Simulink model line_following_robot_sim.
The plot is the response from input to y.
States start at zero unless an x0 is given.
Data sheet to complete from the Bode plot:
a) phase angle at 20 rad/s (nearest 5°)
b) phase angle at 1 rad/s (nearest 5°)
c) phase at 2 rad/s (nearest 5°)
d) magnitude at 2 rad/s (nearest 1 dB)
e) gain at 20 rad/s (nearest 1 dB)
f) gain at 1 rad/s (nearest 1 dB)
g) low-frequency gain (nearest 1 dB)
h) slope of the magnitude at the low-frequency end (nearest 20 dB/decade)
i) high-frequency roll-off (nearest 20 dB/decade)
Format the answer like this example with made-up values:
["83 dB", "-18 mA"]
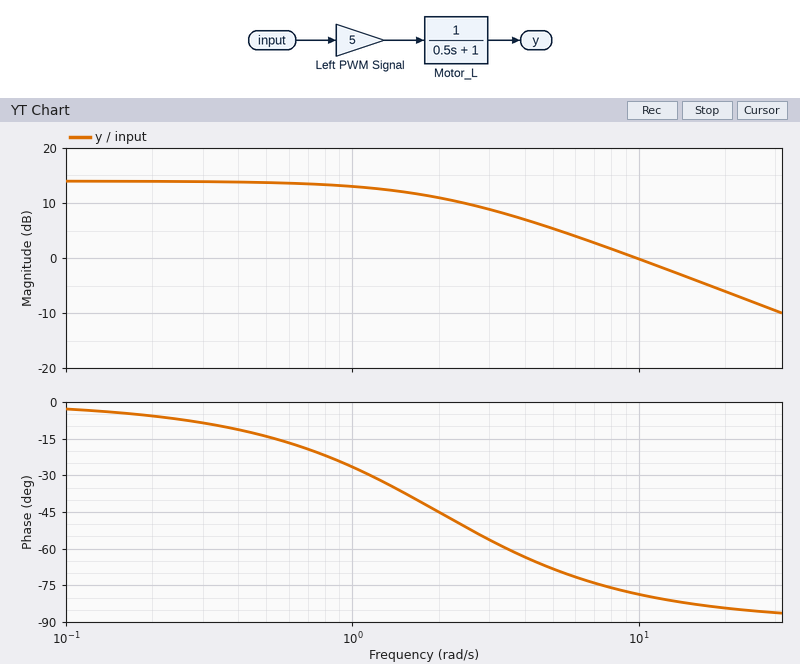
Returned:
["-85°", "-25°", "-45°", "11 dB", "-6 dB", "13 dB", "14 dB", "0 dB/decade", "-20 dB/decade"]
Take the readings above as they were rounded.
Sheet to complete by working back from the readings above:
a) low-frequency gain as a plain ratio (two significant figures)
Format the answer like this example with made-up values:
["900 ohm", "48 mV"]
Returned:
["5.0"]
